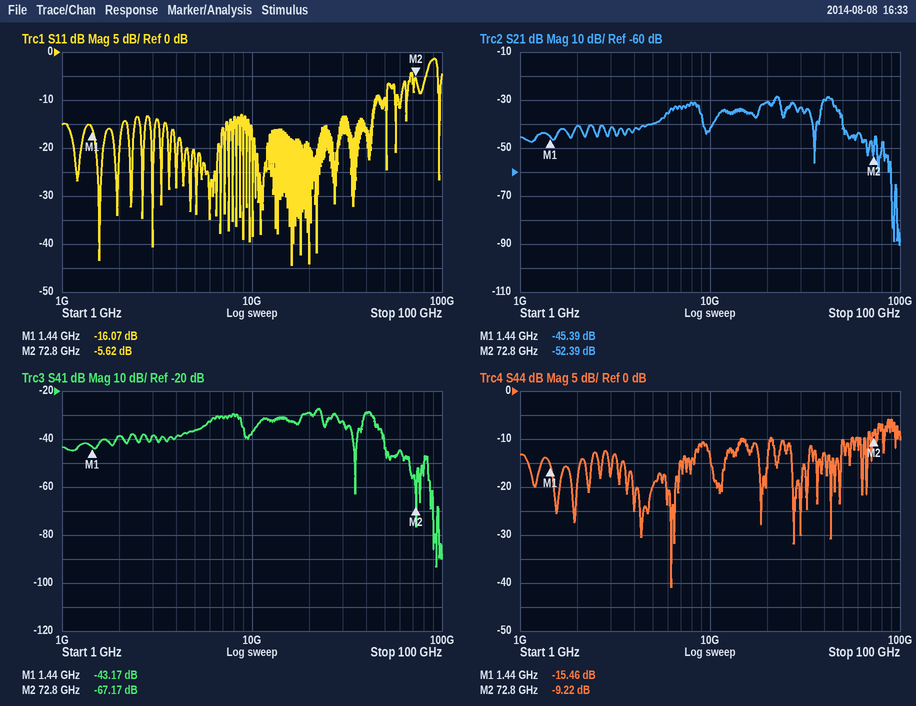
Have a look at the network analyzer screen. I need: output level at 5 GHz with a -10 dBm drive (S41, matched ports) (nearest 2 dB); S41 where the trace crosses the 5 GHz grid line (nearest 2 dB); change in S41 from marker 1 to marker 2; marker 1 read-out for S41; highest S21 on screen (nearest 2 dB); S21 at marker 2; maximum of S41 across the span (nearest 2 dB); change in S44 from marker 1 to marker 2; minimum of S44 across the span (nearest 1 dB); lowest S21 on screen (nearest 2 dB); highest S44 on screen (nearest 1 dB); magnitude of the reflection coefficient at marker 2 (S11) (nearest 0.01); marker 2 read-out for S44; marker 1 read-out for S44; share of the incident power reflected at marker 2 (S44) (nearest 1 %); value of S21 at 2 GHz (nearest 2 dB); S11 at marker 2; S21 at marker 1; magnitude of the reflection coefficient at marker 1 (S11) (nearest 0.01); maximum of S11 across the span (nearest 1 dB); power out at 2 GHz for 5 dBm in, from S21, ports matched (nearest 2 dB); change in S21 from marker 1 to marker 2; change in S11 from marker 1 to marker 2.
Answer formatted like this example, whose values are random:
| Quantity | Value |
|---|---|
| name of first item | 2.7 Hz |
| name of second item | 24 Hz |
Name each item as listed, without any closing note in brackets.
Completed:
| Quantity | Value |
|---|---|
| output level at 5 GHz with a -10 dBm drive (S41, matched ports) | -46 dBm |
| S41 where the trace crosses the 5 GHz grid line | -36 dB |
| change in S41 from marker 1 to marker 2 | -24.00 dB |
| marker 1 read-out for S41 | -43.17 dB |
| highest S21 on screen | -28 dB |
| S21 at marker 2 | -52.39 dB |
| maximum of S41 across the span | -28 dB |
| change in S44 from marker 1 to marker 2 | 6.24 dB |
| minimum of S44 across the span | -41 dB |
| lowest S21 on screen | -90 dB |
| highest S44 on screen | -6 dB |
| magnitude of the reflection coefficient at marker 2 (S11) | 0.52 |
| marker 2 read-out for S44 | -9.22 dB |
| marker 1 read-out for S44 | -15.46 dB |
| share of the incident power reflected at marker 2 (S44) | 12 % |
| value of S21 at 2 GHz | -40 dB |
| S11 at marker 2 | -5.62 dB |
| S21 at marker 1 | -45.39 dB |
| magnitude of the reflection coefficient at marker 1 (S11) | 0.16 |
| maximum of S11 across the span | -1 dB |
| power out at 2 GHz for 5 dBm in, from S21, ports matched | -36 dBm |
| change in S21 from marker 1 to marker 2 | -7.00 dB |
| change in S11 from marker 1 to marker 2 | 10.45 dB |
